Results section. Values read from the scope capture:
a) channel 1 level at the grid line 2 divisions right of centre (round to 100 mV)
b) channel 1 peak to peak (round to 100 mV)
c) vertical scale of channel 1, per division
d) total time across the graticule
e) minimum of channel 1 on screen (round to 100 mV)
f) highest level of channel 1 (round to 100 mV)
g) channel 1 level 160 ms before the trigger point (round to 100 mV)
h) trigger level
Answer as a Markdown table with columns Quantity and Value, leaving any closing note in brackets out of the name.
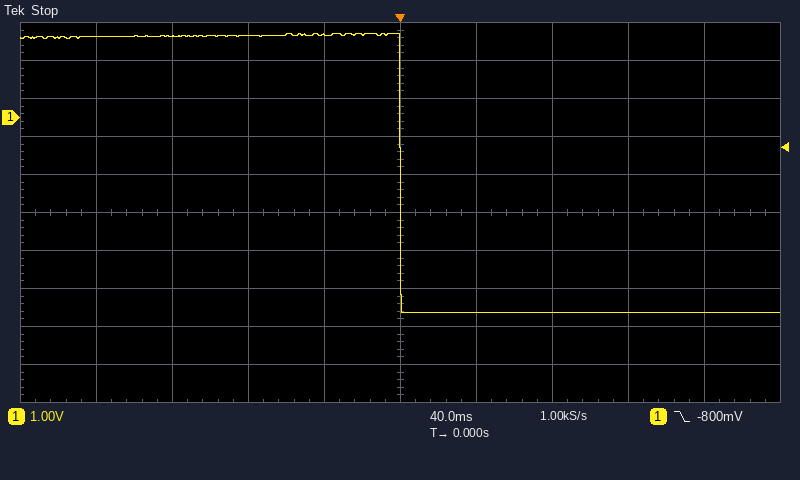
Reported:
| Quantity | Value |
|---|---|
| channel 1 level at the grid line 2 divisions right of centre | -5.1 V |
| channel 1 peak to peak | 7.3 V |
| vertical scale of channel 1, per division | 1 V |
| total time across the graticule | 400 ms |
| minimum of channel 1 on screen | -5.1 V |
| highest level of channel 1 | 2.2 V |
| channel 1 level 160 ms before the trigger point | 2.1 V |
| trigger level | -800 mV |
